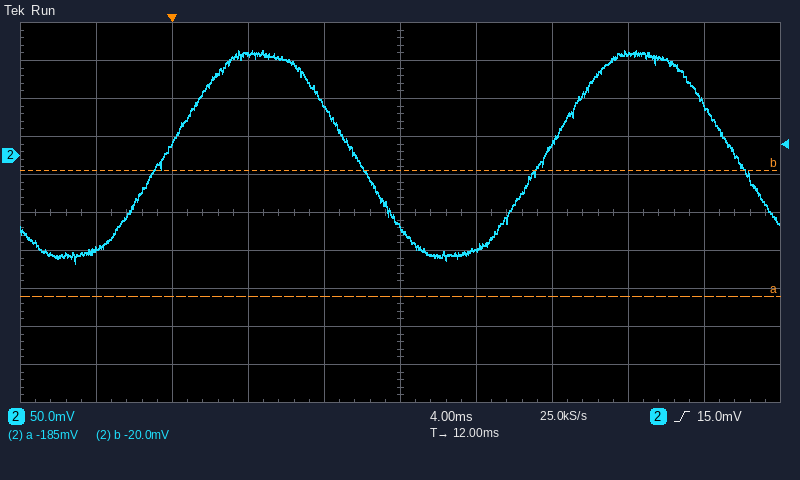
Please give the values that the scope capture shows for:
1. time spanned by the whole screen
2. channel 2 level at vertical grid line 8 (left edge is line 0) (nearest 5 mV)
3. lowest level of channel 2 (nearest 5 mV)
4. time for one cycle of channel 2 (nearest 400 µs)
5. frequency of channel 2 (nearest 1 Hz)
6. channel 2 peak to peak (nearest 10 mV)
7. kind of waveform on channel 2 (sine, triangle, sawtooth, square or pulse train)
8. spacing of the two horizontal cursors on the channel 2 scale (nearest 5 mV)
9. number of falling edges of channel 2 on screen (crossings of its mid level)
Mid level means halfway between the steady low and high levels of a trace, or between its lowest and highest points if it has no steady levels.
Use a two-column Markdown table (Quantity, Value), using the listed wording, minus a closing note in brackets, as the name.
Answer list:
| Quantity | Value |
|---|---|
| time spanned by the whole screen | 40 ms |
| channel 2 level at vertical grid line 8 (left edge is line 0) | 135 mV |
| lowest level of channel 2 | -140 mV |
| time for one cycle of channel 2 | 20.0 ms |
| frequency of channel 2 | 50 Hz |
| channel 2 peak to peak | 280 mV |
| kind of waveform on channel 2 | sine |
| spacing of the two horizontal cursors on the channel 2 scale | 165 mV |
| number of falling edges of channel 2 on screen | 2 |
